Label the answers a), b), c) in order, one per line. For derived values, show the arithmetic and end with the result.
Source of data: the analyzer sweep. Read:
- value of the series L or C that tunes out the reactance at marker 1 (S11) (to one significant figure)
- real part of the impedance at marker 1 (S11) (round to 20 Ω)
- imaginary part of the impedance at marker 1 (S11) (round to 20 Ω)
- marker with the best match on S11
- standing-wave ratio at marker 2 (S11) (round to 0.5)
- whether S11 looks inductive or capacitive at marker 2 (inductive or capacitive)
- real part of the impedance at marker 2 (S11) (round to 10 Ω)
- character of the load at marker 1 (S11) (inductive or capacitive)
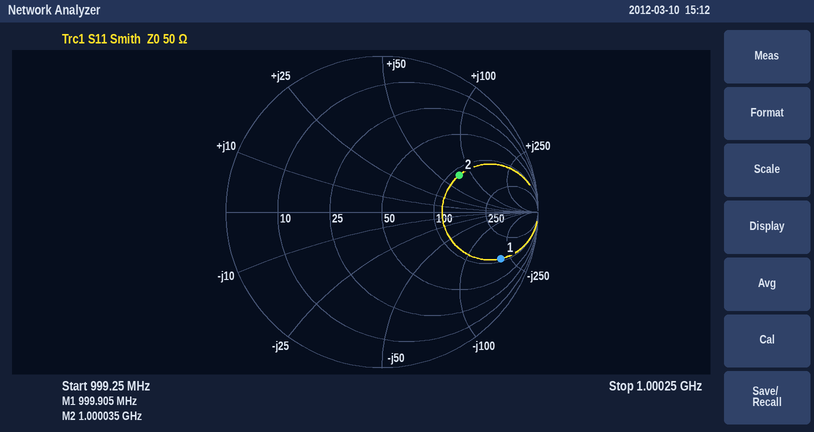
a) L = 200 Ω/(2π × 999.905 MHz) ≈ 31.8 nH, so 30 nH to one significant figure
b) 120 Ω
c) -200 Ω
d) marker 2
e) 3.5
f) inductive
g) 110 Ω
h) capacitive
